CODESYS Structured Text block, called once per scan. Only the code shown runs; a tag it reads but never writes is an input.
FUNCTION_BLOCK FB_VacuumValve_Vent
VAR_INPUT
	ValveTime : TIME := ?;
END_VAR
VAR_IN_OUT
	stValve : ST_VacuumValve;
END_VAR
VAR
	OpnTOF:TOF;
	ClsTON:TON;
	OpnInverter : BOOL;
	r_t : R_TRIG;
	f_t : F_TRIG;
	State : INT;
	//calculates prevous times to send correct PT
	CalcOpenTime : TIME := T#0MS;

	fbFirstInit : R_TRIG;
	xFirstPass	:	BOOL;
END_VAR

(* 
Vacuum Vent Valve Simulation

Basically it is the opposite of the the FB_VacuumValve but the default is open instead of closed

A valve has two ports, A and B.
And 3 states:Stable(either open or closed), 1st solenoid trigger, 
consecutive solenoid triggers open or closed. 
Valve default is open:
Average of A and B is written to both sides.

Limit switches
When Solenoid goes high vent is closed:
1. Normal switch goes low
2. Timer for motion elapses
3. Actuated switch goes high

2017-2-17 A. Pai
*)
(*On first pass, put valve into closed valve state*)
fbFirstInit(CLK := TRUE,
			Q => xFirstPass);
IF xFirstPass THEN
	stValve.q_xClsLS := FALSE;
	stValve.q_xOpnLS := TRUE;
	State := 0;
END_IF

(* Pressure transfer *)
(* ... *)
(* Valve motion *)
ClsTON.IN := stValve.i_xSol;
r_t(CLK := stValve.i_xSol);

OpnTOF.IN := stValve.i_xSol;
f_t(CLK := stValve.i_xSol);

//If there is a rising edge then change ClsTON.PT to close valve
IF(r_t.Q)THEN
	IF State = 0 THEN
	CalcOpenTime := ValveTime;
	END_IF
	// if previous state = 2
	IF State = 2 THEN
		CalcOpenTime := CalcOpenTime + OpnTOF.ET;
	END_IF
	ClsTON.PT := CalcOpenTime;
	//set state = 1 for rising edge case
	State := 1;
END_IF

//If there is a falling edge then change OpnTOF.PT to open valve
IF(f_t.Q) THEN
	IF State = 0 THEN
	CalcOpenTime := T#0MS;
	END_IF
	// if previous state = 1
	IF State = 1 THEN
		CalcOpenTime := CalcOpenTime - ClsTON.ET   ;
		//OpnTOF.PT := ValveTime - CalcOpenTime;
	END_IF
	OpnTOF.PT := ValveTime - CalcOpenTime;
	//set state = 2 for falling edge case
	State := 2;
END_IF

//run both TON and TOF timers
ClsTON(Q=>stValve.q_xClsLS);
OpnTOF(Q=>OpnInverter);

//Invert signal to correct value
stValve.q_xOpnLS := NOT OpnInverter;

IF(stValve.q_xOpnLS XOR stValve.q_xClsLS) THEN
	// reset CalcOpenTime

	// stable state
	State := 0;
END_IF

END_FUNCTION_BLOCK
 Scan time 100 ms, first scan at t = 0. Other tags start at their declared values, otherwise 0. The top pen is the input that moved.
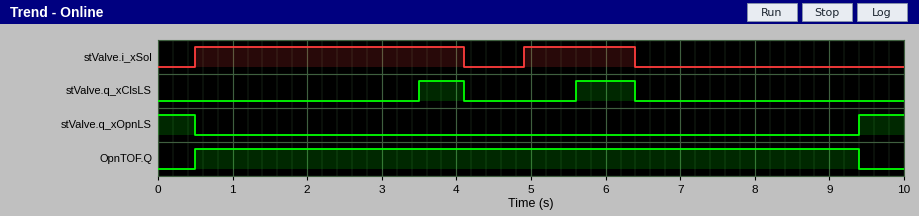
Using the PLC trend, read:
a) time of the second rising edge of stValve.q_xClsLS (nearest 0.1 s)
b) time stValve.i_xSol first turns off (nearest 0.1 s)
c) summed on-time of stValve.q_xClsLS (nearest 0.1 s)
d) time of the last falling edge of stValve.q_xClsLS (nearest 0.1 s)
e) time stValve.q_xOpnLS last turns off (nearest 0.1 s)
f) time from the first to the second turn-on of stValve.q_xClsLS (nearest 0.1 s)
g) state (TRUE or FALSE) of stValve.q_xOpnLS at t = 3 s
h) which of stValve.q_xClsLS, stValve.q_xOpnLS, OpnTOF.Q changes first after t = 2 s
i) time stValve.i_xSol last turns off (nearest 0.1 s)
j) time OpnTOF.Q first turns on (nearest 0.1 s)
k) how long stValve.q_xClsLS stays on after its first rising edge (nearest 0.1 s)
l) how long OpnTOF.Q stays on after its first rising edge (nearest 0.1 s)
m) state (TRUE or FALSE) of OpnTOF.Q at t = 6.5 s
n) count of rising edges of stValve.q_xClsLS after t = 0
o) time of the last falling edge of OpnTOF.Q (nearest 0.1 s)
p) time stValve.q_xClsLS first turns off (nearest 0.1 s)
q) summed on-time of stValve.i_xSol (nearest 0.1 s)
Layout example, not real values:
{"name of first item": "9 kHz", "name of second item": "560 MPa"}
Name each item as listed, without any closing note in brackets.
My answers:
{"time of the second rising edge of stValve.q_xClsLS": "5.6 s", "time stValve.i_xSol first turns off": "4.1 s", "summed on-time of stValve.q_xClsLS": "1.4 s", "time of the last falling edge of stValve.q_xClsLS": "6.4 s", "time stValve.q_xOpnLS last turns off": "0.5 s", "time from the first to the second turn-on of stValve.q_xClsLS": "2.1 s", "state (TRUE or FALSE) of stValve.q_xOpnLS at t = 3 s": "FALSE", "which of stValve.q_xClsLS, stValve.q_xOpnLS, OpnTOF.Q changes first after t = 2 s": "stValve.q_xClsLS", "time stValve.i_xSol last turns off": "6.4 s", "time OpnTOF.Q first turns on": "0.5 s", "how long stValve.q_xClsLS stays on after its first rising edge": "0.6 s", "how long OpnTOF.Q stays on after its first rising edge": "8.9 s", "state (TRUE or FALSE) of OpnTOF.Q at t = 6.5 s": "TRUE", "count of rising edges of stValve.q_xClsLS after t = 0": "2", "time of the last falling edge of OpnTOF.Q": "9.4 s", "time stValve.q_xClsLS first turns off": "4.1 s", "summed on-time of stValve.i_xSol": "5.1 s"}
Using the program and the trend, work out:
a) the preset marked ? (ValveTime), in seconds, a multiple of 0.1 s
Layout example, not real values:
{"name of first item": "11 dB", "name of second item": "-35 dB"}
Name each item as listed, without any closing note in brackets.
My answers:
{"the preset marked ? (ValveTime), in seconds, a multiple of 0.1 s": "3.0 s"}
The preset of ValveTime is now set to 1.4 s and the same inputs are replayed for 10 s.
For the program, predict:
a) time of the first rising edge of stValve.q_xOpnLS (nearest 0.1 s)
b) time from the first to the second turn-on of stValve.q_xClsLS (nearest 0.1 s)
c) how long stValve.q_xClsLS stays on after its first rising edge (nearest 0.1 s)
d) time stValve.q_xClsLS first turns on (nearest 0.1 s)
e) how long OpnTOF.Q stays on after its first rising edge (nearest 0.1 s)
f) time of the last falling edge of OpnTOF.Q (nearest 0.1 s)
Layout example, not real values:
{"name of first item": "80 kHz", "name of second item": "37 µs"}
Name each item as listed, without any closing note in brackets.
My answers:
{"time of the first rising edge of stValve.q_xOpnLS": "7.8 s", "time from the first to the second turn-on of stValve.q_xClsLS": "3.7 s", "how long stValve.q_xClsLS stays on after its first rising edge": "2.2 s", "time stValve.q_xClsLS first turns on": "1.9 s", "how long OpnTOF.Q stays on after its first rising edge": "7.3 s", "time of the last falling edge of OpnTOF.Q": "7.8 s"}
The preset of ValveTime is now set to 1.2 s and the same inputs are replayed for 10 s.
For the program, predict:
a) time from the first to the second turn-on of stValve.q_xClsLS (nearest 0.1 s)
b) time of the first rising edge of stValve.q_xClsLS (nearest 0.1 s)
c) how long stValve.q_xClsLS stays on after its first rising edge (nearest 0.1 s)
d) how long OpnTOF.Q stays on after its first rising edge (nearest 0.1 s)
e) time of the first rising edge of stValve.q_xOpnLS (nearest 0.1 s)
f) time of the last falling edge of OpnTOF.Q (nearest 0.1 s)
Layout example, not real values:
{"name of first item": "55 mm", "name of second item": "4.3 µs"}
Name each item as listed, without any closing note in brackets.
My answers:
{"time from the first to the second turn-on of stValve.q_xClsLS": "3.9 s", "time of the first rising edge of stValve.q_xClsLS": "1.7 s", "how long stValve.q_xClsLS stays on after its first rising edge": "2.4 s", "how long OpnTOF.Q stays on after its first rising edge": "7.1 s", "time of the first rising edge of stValve.q_xOpnLS": "7.6 s", "time of the last falling edge of OpnTOF.Q": "7.6 s"}
